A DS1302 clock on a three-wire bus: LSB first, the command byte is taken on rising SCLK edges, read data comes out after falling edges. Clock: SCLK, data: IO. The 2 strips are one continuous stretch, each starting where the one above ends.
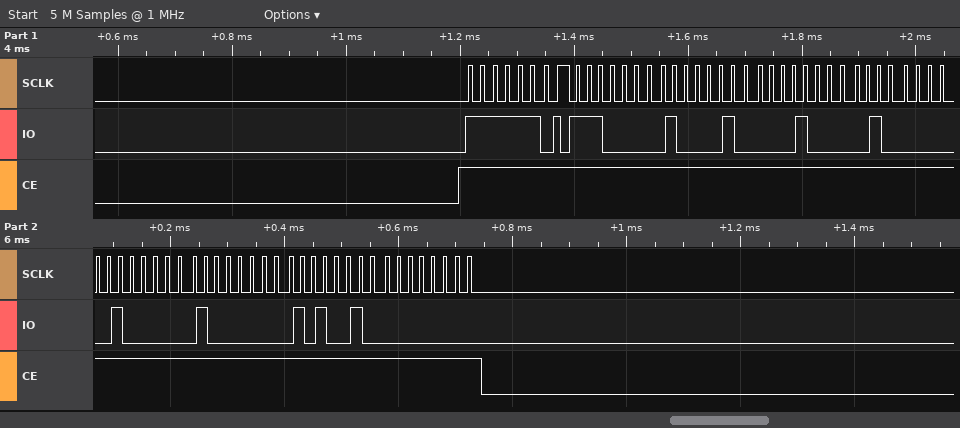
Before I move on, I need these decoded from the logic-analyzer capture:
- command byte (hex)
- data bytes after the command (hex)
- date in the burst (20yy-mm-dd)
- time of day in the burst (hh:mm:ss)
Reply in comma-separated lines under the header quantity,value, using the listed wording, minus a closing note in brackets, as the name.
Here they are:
quantity,value
command byte,0xBF
data bytes after the command,07 21 08 02 02 01 25 00
date in the burst,2025-02-02
time of day in the burst,08:21:07
